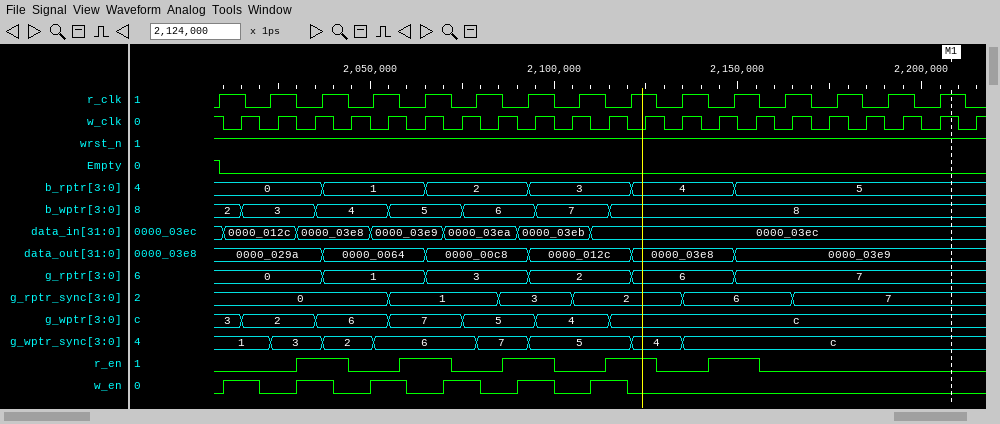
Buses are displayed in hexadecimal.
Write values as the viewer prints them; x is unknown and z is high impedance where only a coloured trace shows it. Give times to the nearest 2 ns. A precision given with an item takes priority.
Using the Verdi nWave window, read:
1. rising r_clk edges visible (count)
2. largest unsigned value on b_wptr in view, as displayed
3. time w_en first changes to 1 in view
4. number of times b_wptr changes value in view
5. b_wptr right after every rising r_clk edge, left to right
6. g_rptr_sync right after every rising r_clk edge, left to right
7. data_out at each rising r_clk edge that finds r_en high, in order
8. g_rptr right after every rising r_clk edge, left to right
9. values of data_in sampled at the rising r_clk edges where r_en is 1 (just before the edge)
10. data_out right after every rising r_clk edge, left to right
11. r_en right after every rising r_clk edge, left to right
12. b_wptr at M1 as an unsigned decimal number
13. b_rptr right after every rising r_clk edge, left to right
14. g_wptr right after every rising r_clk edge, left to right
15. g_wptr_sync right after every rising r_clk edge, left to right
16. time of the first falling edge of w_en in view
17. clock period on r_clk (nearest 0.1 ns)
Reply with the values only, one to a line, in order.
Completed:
15
8
2010 ns
6
2, 3, 4, 4, 5, 6, 6, 7, 8, 8, 8, 8, 8, 8, 8
0, 0, 0, 0, 1, 1, 3, 2, 2, 6, 6, 6, 7, 7, 7
0000_029a, 0000_0064, 0000_00c8, 0000_012c, 0000_03e8
0, 0, 1, 1, 3, 3, 2, 2, 6, 6, 7, 7, 7, 7, 7
0000_03e8, 0000_03e9, 0000_03eb, 0000_03ec, 0000_03ec
0000_029a, 0000_029a, 0000_0064, 0000_0064, 0000_00c8, 0000_00c8, 0000_012c, 0000_012c, 0000_03e8, 0000_03e8, 0000_03e9, 0000_03e9, 0000_03e9, 0000_03e9, 0000_03e9
0 0 1 0 1 0 1 0 1 0 1 0 0 0 0
8
0, 0, 1, 1, 2, 2, 3, 3, 4, 4, 5, 5, 5, 5, 5
3, 2, 6, 6, 7, 5, 5, 4, c, c, c, c, c, c, c
1, 3, 2, 6, 6, 7, 5, 5, 4, c, c, c, c, c, c
2020 ns
14 ns
